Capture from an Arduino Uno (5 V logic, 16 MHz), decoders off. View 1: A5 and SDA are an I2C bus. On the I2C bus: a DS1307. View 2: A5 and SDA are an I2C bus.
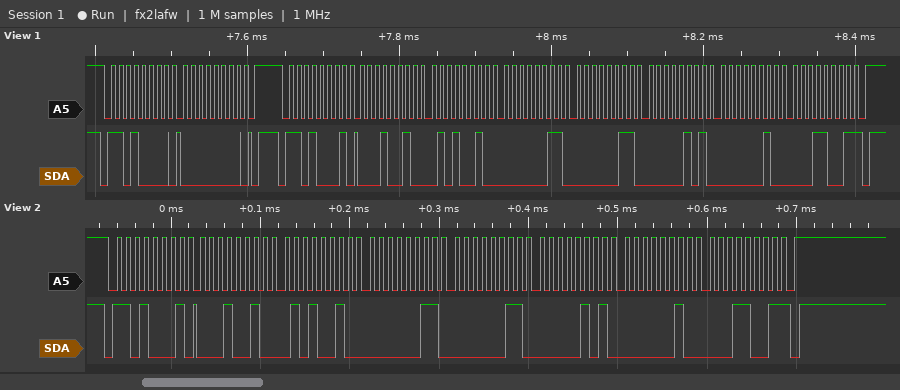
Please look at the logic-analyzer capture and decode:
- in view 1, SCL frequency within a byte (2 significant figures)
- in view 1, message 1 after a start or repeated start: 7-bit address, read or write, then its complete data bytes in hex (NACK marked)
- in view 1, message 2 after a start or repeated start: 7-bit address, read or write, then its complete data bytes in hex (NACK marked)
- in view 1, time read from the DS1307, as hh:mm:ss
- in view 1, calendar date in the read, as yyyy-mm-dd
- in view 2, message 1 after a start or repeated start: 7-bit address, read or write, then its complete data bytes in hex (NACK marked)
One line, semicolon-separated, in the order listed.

100 kHz; 0x68 write: 00; 0x68 read: 12 52 03 03 05 02 19 NACK; 03:52:12; 2019-02-05; 0x68 read: 12 52 03 03 05 02 19 NACK
